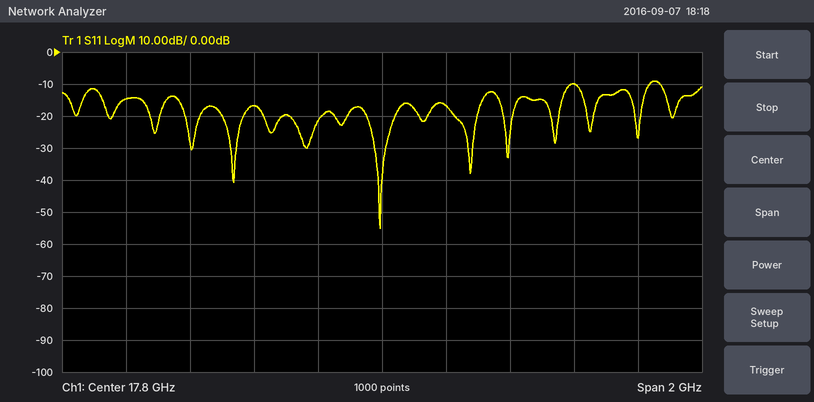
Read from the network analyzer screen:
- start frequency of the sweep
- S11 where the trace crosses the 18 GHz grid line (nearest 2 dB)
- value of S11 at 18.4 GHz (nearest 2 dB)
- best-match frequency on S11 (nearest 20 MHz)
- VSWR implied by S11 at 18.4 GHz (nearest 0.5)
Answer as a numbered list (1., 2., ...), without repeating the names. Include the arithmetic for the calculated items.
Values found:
1. 16.8 GHz
2. -16 dB
3. -10 dB
4. 17.80 GHz
5. |Γ| = 10^(-10/20) = 0.3162; VSWR = (1 + 0.3162)/(1 − 0.3162) ≈ 1.92, so 2.0 to the nearest 0.5
